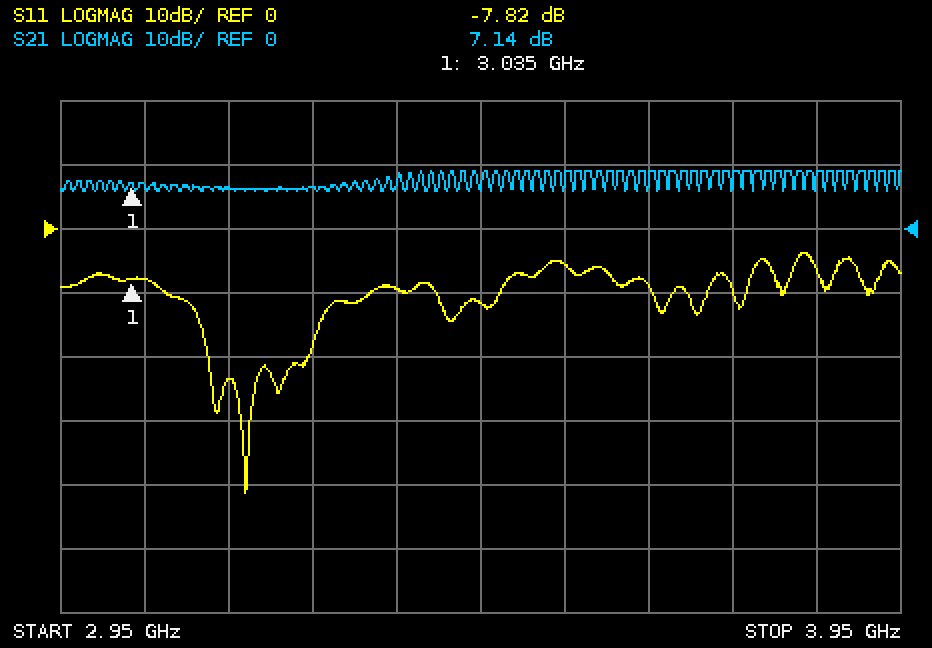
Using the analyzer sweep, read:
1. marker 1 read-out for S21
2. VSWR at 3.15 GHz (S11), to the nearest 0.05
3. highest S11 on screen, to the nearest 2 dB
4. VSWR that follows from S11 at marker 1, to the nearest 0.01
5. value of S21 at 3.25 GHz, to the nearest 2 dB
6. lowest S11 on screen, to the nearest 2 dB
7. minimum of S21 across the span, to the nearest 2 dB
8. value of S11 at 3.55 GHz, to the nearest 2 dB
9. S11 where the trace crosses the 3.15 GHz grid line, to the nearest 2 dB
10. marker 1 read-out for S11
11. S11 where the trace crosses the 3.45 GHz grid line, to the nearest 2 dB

7.14 dB
1.15
-4 dB
2.37
6 dB
-42 dB
6 dB
-6 dB
-24 dB
-7.82 dB
-12 dB
